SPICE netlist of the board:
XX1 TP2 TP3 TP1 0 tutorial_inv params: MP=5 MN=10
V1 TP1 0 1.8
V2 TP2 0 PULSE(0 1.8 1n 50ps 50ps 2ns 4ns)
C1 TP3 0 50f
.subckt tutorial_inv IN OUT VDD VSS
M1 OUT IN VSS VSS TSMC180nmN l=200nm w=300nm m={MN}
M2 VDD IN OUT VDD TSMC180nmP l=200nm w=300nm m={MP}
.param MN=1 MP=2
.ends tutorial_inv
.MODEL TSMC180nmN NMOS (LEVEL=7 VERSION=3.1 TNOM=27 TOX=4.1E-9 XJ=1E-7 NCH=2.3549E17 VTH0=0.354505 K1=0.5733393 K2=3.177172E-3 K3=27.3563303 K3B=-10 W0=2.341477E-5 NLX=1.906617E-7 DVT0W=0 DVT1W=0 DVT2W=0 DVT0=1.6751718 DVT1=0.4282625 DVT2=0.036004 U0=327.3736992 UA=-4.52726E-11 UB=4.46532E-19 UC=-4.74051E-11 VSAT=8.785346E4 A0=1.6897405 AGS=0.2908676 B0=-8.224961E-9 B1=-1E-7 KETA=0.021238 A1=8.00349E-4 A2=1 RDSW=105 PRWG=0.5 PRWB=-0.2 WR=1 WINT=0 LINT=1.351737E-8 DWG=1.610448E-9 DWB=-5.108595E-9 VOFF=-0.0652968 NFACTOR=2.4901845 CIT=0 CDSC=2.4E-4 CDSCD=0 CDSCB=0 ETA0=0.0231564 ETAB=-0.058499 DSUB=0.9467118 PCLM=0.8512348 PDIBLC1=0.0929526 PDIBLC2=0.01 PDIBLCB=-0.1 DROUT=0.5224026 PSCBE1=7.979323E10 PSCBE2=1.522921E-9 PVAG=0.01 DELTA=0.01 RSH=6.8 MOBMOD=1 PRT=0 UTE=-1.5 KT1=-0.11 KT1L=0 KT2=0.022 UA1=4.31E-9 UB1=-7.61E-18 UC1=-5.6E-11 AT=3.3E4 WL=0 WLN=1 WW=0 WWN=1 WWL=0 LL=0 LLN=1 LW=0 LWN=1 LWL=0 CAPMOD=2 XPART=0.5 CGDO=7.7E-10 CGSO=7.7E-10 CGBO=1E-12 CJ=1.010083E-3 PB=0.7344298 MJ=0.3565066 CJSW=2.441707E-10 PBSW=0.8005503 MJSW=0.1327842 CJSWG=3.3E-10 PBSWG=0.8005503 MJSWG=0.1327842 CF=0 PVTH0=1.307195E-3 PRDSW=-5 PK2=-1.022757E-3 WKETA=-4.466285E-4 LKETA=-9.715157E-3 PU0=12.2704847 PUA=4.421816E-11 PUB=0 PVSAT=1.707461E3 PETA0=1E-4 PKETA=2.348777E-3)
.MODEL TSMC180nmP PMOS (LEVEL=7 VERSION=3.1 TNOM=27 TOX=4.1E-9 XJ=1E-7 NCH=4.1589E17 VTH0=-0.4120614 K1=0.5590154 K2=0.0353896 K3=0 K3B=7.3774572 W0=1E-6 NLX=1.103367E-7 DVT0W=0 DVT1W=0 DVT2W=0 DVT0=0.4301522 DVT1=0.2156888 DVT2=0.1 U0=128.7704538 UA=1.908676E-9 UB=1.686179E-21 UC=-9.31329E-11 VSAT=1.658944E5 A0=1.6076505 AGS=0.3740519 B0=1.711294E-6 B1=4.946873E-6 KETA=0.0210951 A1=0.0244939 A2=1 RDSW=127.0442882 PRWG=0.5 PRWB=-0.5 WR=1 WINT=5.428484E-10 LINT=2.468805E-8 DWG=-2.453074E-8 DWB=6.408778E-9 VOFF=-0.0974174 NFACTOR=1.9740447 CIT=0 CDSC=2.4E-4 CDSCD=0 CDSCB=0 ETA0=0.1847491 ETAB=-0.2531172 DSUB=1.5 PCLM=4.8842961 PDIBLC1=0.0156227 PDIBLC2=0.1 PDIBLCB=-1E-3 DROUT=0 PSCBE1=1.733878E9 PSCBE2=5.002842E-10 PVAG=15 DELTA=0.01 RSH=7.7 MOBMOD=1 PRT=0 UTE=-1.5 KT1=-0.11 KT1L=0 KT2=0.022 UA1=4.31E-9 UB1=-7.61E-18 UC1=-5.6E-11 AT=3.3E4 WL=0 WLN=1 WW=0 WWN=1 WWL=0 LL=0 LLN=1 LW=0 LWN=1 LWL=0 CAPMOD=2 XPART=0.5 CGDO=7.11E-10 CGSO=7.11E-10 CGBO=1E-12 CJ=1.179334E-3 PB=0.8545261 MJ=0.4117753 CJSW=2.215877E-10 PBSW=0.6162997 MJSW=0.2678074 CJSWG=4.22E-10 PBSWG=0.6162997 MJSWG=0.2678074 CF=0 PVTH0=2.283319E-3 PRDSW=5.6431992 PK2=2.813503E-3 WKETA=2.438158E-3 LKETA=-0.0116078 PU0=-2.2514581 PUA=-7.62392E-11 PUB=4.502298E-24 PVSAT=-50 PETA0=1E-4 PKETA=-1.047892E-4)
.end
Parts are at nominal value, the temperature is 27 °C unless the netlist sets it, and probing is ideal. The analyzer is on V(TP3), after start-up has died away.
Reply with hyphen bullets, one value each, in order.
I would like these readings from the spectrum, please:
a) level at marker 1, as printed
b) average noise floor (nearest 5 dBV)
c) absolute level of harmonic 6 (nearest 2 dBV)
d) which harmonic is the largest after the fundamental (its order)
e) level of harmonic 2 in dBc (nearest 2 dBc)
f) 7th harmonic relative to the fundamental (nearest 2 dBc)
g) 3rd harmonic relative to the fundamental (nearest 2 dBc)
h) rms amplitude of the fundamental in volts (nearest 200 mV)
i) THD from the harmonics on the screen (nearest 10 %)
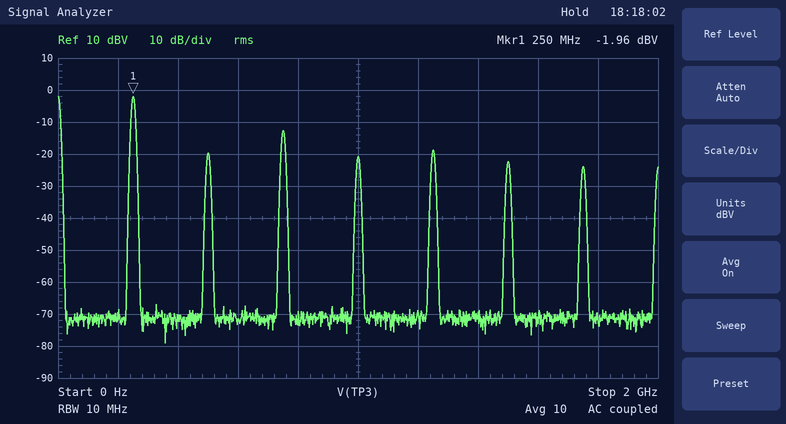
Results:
- -1.96 dBV
- -70 dBV
- -22 dBV
- 3
- -18 dBc
- -22 dBc
- -10 dBc
- 800 mV
- 40 %
